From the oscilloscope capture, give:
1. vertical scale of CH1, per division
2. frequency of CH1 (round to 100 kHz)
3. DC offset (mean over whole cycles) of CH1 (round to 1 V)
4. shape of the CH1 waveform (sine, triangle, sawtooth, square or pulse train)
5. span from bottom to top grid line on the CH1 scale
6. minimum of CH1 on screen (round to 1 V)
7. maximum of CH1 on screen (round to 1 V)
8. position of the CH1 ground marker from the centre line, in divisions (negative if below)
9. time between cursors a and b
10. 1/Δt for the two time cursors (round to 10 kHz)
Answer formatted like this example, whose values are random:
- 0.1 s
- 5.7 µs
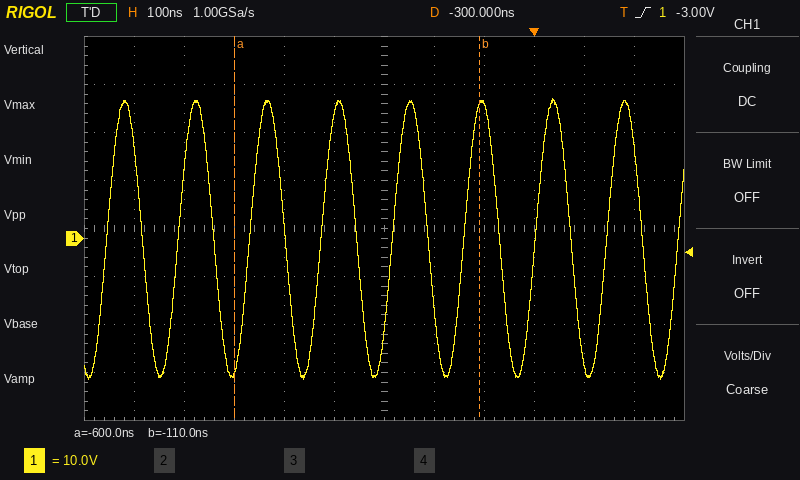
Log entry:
- 10 V
- 7.0 MHz
- 0 V
- sine
- 80 V
- -29 V
- 29 V
- -0.2 div
- 490 ns
- 2.04 MHz
